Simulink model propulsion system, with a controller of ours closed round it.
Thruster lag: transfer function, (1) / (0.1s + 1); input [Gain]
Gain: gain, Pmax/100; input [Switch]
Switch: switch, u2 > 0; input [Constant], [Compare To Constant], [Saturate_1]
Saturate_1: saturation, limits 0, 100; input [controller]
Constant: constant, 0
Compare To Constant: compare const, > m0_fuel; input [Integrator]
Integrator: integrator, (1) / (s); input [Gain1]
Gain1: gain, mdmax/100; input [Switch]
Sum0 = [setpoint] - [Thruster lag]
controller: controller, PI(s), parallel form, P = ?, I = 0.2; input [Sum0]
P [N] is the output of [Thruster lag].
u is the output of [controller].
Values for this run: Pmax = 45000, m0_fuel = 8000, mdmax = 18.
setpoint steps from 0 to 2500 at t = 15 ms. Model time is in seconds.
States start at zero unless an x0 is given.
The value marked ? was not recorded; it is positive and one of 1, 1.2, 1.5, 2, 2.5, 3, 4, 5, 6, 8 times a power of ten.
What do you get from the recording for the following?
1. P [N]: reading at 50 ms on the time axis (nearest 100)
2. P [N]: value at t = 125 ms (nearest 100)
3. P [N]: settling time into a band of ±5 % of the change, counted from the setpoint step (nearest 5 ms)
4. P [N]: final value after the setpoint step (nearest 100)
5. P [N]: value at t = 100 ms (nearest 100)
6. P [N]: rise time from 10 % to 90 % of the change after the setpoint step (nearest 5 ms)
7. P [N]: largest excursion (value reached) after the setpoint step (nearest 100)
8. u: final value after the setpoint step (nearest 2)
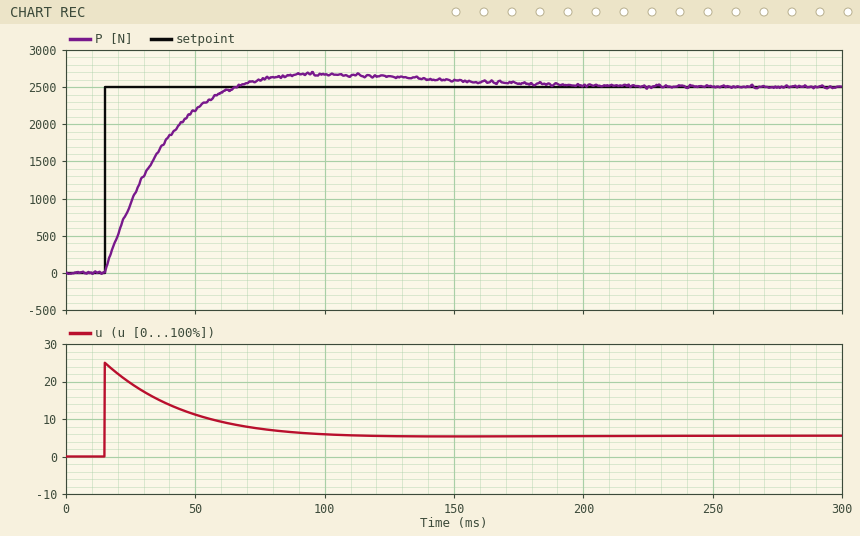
2200
2600
120 ms
2500
2700
35 ms
2700
6
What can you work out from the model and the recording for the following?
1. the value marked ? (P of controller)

0.01
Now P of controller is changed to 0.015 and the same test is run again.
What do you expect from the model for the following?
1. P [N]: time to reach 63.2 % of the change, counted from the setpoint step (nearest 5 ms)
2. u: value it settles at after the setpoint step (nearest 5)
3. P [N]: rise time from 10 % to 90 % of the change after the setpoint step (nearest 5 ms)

15 ms
5
30 ms
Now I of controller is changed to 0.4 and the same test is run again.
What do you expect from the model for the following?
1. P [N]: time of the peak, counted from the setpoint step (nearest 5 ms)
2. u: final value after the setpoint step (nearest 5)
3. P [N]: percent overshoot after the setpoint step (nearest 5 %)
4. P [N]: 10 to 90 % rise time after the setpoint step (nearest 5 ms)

60 ms
5
15 %
25 ms
